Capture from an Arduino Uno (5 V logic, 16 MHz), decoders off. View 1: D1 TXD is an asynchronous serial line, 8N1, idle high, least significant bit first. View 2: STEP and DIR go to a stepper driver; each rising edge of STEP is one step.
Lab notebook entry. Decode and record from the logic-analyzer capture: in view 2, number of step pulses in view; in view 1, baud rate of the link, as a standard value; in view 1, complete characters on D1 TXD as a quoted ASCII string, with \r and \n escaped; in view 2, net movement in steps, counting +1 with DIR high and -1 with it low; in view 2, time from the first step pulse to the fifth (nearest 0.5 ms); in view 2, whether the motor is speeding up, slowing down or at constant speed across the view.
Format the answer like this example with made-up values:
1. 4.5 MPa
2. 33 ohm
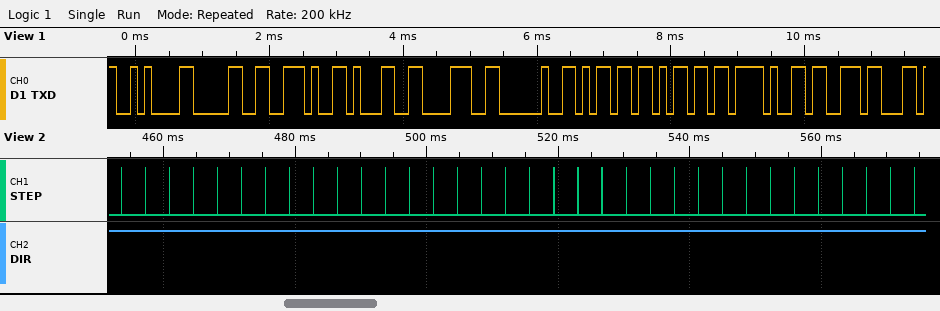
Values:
1. 34
2. 9600 baud
3. "\n0.18 mm/s"
4. +34
5. 14.5 ms
6. constant speed
